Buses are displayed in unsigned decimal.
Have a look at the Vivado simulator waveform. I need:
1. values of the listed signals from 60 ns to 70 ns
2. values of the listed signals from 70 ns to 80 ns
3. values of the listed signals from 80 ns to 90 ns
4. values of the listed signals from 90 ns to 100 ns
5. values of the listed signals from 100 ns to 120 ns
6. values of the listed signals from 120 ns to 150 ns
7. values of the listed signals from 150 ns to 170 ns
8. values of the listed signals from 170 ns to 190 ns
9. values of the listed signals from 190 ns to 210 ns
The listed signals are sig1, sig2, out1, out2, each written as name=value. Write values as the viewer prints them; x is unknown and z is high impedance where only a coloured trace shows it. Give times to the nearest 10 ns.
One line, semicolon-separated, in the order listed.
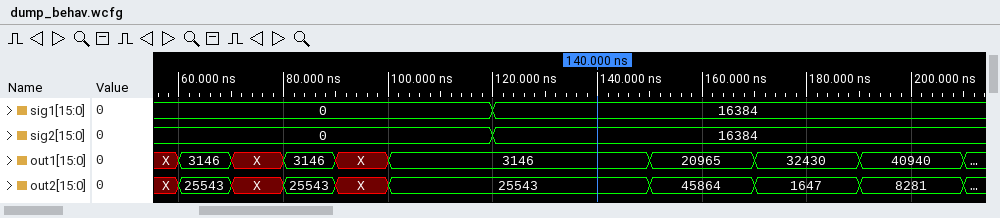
sig1=0, sig2=0, out1=3146, out2=25543; sig1=0, sig2=0, out1=X, out2=X; sig1=0, sig2=0, out1=3146, out2=25543; sig1=0, sig2=0, out1=X, out2=X; sig1=0, sig2=0, out1=3146, out2=25543; sig1=16384, sig2=16384, out1=3146, out2=25543; sig1=16384, sig2=16384, out1=20965, out2=45864; sig1=16384, sig2=16384, out1=32430, out2=1647; sig1=16384, sig2=16384, out1=40940, out2=8281
